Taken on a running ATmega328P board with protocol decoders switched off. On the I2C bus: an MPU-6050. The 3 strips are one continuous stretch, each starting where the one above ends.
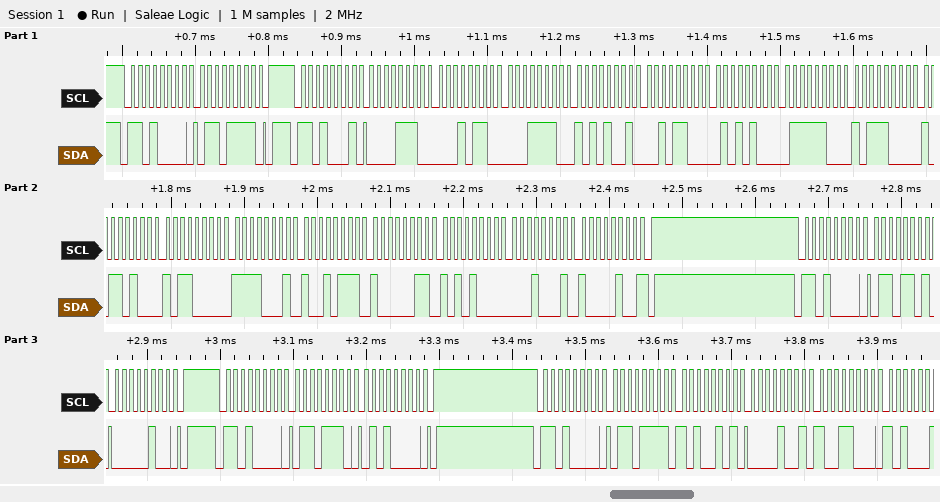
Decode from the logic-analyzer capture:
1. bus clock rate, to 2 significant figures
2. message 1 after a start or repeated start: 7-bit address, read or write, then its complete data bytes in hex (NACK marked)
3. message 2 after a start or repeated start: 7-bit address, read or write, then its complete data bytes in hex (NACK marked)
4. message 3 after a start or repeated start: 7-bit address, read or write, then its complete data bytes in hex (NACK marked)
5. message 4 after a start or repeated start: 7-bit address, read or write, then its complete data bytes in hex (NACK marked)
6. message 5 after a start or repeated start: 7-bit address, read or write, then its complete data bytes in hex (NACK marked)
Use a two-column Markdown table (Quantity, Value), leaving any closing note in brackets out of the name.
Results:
| Quantity | Value |
|---|---|
| bus clock rate, to 2 significant figures | 100 kHz |
| message 1 after a start or repeated start: 7-bit address, read or write, then its complete data bytes in hex | 0x68 write: 6F |
| message 2 after a start or repeated start: 7-bit address, read or write, then its complete data bytes in hex | 0x68 read: 0E 16 1E A9 2C 54 7C B8 B4 B0 F1 97 83 A8 11 84 NACK |
| message 3 after a start or repeated start: 7-bit address, read or write, then its complete data bytes in hex | 0x68 write: 6D 04 |
| message 4 after a start or repeated start: 7-bit address, read or write, then its complete data bytes in hex | 0x68 write: 6E 50 |
| message 5 after a start or repeated start: 7-bit address, read or write, then its complete data bytes in hex | 0x68 write: 6F A5 09 98 |
